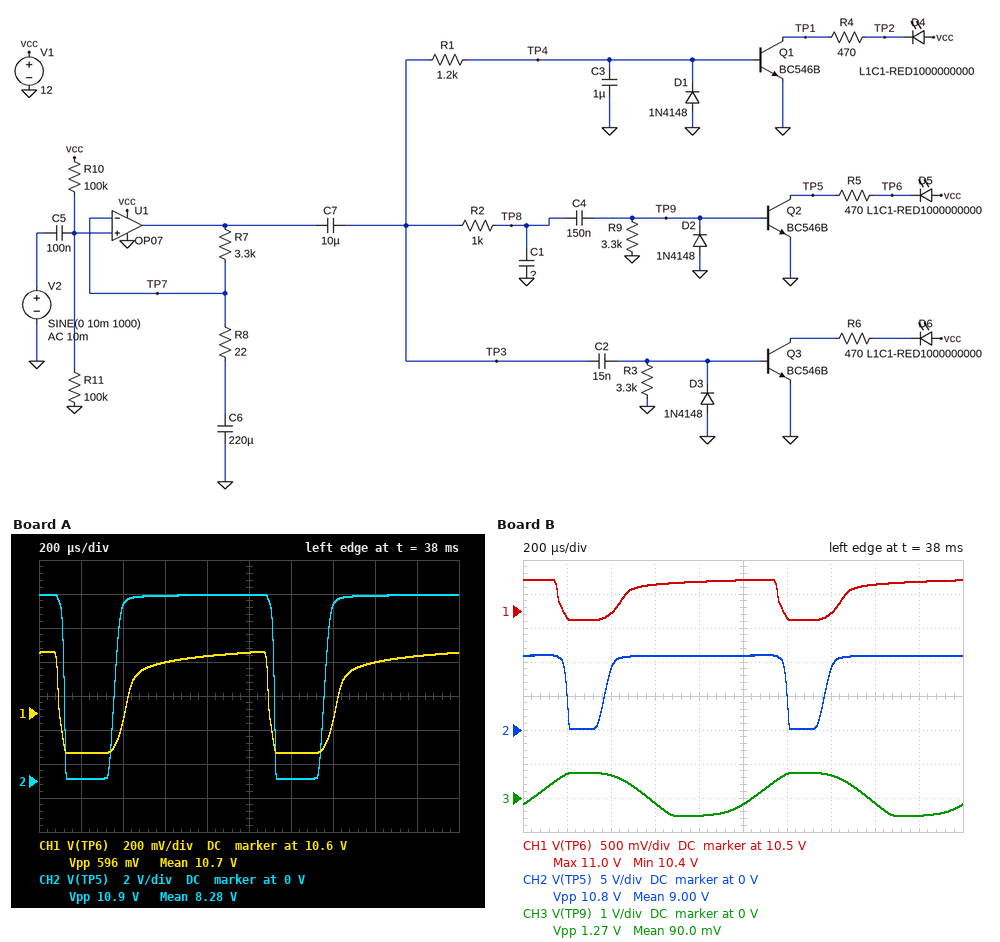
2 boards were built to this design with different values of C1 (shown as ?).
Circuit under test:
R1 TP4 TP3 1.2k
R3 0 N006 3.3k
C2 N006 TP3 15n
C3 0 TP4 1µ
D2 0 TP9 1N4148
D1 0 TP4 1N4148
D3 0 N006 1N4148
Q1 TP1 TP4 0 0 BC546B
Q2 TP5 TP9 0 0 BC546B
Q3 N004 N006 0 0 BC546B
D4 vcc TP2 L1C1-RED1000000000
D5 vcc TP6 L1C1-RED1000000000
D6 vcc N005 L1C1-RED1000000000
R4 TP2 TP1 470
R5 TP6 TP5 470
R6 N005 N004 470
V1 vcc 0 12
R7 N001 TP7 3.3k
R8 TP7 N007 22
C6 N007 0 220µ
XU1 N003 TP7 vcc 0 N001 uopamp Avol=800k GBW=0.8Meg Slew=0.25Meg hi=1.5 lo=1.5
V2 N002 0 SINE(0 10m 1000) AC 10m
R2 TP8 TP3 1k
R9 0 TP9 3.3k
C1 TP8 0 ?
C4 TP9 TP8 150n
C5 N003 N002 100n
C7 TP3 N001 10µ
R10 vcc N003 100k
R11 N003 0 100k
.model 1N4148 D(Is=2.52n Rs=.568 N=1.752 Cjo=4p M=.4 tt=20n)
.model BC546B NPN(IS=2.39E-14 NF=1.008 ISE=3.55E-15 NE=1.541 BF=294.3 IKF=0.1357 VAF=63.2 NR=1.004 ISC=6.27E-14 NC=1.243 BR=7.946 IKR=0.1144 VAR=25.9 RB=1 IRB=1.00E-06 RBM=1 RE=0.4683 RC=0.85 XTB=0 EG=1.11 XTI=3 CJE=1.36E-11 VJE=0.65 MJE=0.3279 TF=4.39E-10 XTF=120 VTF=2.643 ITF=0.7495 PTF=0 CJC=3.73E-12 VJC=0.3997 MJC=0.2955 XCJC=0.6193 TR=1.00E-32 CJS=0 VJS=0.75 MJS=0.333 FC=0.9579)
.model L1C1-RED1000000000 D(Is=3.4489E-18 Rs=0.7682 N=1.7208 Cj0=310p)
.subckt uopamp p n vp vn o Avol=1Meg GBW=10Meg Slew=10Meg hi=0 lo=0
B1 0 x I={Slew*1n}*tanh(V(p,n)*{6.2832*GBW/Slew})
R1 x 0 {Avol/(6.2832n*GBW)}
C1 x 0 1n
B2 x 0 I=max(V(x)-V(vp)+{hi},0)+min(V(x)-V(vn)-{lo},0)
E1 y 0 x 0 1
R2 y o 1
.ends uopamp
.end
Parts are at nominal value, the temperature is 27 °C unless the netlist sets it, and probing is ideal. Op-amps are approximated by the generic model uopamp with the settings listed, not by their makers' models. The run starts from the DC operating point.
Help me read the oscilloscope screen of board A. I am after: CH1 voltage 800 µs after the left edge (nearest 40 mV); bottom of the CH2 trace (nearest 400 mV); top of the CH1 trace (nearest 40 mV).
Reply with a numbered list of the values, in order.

1. 10.92 V
2. 0 V
3. 10.96 V
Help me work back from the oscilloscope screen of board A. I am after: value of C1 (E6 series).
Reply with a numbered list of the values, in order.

1. 68 nF
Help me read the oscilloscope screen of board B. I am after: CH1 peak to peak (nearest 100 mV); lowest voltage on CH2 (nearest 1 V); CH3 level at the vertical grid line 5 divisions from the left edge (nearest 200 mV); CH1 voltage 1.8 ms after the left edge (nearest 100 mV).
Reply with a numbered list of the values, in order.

1. 600 mV
2. 0 V
3. -200 mV
4. 10.9 V
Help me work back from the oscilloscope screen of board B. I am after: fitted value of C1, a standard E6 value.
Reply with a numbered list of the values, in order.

1. 150 nF
